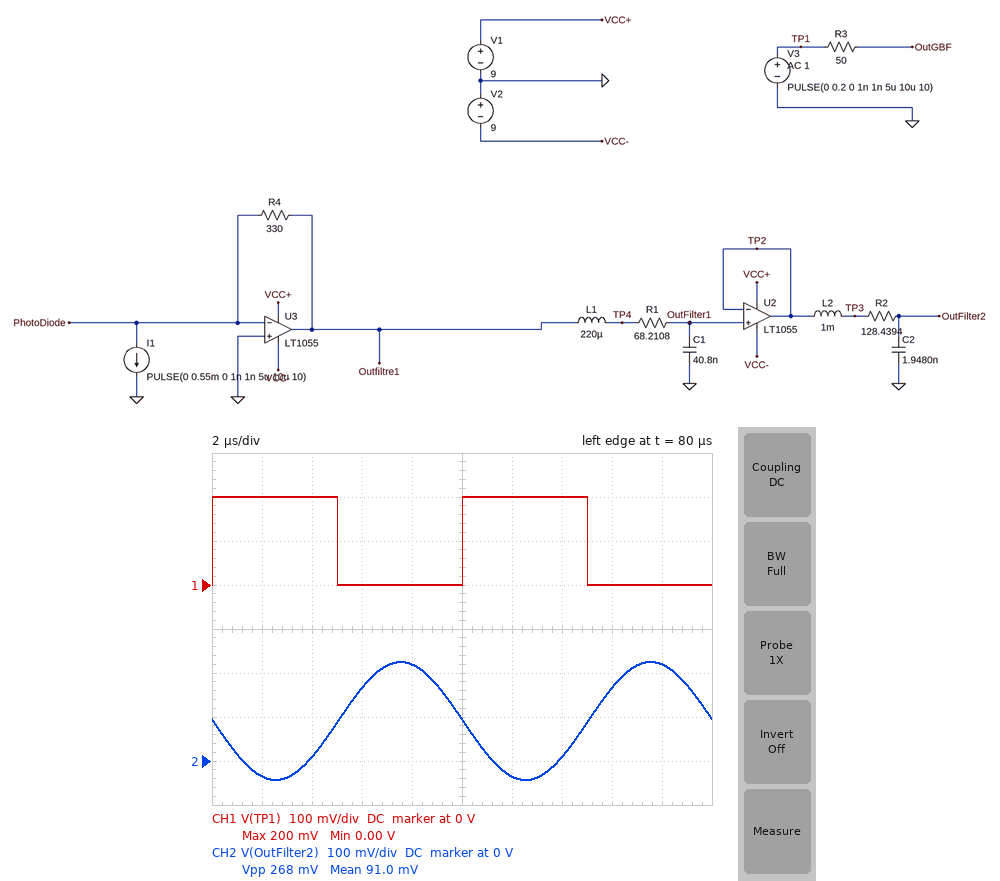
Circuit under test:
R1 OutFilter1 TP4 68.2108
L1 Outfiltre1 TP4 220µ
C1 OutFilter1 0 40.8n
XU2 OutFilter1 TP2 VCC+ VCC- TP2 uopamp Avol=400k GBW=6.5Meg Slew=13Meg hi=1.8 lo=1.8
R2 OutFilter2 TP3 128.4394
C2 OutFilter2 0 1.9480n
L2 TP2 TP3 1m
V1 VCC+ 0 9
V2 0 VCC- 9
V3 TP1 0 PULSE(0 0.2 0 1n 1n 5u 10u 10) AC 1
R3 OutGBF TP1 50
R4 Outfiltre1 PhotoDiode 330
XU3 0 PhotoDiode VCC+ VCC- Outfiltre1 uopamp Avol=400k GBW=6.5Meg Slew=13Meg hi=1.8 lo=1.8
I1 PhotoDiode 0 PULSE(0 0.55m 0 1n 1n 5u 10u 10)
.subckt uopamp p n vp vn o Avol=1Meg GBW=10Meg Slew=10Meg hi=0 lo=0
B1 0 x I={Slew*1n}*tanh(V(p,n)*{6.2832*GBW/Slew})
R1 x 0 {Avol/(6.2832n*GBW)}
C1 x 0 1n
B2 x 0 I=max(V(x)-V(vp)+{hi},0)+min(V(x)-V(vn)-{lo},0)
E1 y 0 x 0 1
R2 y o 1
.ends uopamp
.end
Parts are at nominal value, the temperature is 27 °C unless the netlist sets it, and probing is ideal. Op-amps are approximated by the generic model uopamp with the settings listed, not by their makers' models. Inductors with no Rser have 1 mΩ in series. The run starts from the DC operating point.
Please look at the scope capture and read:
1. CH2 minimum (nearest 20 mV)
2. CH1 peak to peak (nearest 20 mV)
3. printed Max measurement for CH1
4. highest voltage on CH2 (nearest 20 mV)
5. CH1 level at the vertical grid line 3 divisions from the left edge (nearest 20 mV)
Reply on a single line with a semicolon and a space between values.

-40 mV; 200 mV; 200 mV; 220 mV; 0 V
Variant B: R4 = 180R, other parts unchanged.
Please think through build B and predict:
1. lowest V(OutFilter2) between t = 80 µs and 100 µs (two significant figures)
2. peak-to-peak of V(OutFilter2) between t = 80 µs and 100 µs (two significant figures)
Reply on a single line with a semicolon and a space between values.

-24 mV; 150 mV
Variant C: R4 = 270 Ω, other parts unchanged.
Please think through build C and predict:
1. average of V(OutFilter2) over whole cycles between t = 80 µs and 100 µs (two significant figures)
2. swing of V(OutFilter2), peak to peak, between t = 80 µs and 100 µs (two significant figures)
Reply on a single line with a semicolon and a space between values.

74 mV; 220 mV
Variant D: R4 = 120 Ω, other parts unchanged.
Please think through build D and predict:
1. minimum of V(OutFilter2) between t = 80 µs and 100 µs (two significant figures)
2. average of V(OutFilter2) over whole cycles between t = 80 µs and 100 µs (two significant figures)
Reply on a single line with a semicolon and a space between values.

-16 mV; 33 mV
